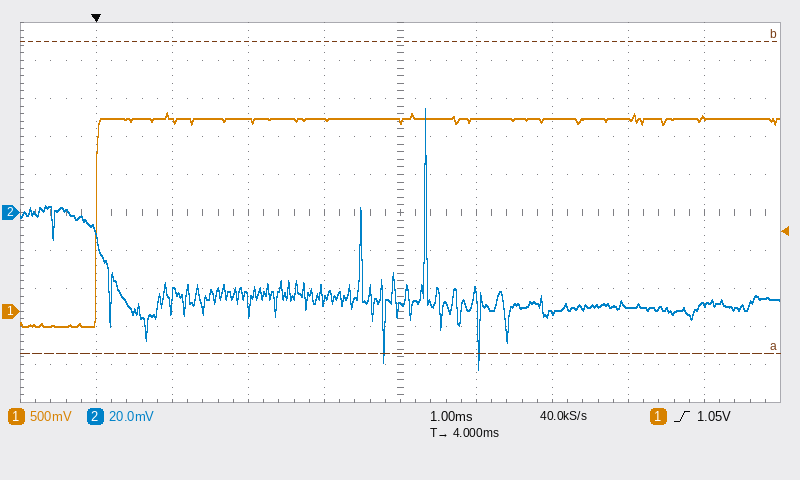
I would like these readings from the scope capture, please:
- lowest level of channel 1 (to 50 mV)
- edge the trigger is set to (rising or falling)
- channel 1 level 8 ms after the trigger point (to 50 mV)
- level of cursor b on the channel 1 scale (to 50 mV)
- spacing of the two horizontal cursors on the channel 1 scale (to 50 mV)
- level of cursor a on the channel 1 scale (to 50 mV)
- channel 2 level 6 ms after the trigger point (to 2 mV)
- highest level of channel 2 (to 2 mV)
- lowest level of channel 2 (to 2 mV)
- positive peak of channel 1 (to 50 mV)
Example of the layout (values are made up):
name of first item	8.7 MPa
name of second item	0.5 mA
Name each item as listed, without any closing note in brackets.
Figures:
lowest level of channel 1	-200 mV
edge the trigger is set to	rising
channel 1 level 8 ms after the trigger point	2.55 V
level of cursor b on the channel 1 scale	3.55 V
spacing of the two horizontal cursors on the channel 1 scale	4.10 V
level of cursor a on the channel 1 scale	-550 mV
channel 2 level 6 ms after the trigger point	-52 mV
highest level of channel 2	54 mV
lowest level of channel 2	-82 mV
positive peak of channel 1	2.60 V
